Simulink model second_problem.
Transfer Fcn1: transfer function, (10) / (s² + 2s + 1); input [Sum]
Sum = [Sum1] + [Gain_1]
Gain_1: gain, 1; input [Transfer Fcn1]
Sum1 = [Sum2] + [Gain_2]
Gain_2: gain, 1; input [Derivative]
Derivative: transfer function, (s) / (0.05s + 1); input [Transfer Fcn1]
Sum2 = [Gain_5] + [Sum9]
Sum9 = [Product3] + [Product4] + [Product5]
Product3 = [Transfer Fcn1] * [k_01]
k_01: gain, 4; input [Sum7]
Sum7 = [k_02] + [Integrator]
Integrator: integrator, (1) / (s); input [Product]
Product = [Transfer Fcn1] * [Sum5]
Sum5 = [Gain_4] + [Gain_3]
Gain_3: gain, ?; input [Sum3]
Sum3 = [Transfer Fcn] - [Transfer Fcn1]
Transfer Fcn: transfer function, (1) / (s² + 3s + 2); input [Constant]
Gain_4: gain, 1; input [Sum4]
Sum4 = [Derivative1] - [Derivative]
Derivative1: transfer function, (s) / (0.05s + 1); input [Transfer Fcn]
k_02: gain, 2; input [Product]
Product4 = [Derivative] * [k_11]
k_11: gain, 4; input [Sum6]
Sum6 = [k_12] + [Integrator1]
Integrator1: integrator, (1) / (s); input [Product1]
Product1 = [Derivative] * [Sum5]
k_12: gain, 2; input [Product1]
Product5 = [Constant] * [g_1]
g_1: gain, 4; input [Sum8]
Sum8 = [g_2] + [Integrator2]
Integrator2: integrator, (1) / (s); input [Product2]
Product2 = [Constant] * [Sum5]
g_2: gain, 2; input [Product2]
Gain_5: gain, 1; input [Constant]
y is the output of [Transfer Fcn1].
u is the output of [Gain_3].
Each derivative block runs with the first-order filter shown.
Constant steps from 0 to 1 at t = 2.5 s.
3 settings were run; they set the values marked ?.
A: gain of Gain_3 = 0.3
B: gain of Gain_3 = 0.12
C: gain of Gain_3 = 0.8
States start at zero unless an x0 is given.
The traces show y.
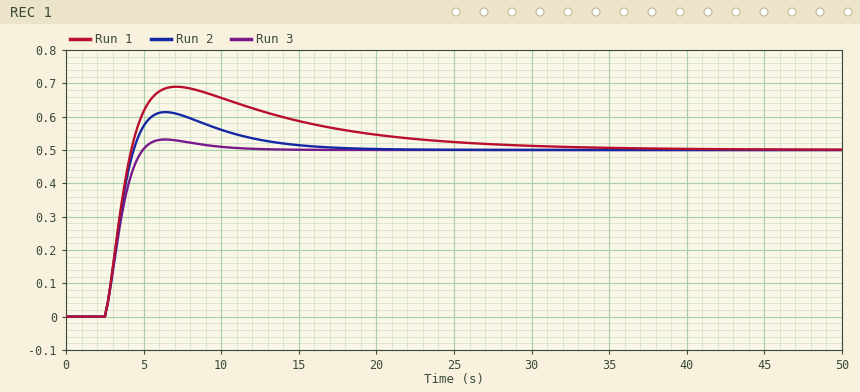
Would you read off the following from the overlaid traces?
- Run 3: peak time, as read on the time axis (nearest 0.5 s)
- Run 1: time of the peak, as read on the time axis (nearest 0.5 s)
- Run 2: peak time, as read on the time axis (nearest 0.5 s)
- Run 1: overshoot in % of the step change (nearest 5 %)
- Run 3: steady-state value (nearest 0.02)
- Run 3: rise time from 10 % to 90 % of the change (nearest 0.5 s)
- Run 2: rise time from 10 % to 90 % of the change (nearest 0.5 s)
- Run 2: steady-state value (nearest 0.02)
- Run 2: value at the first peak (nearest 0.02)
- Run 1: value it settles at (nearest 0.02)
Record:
6.5 s
7.0 s
6.5 s
40 %
0.50
1.5 s
1.5 s
0.50
0.62
0.50
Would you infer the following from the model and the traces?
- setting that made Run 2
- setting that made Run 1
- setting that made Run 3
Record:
A
B
C
